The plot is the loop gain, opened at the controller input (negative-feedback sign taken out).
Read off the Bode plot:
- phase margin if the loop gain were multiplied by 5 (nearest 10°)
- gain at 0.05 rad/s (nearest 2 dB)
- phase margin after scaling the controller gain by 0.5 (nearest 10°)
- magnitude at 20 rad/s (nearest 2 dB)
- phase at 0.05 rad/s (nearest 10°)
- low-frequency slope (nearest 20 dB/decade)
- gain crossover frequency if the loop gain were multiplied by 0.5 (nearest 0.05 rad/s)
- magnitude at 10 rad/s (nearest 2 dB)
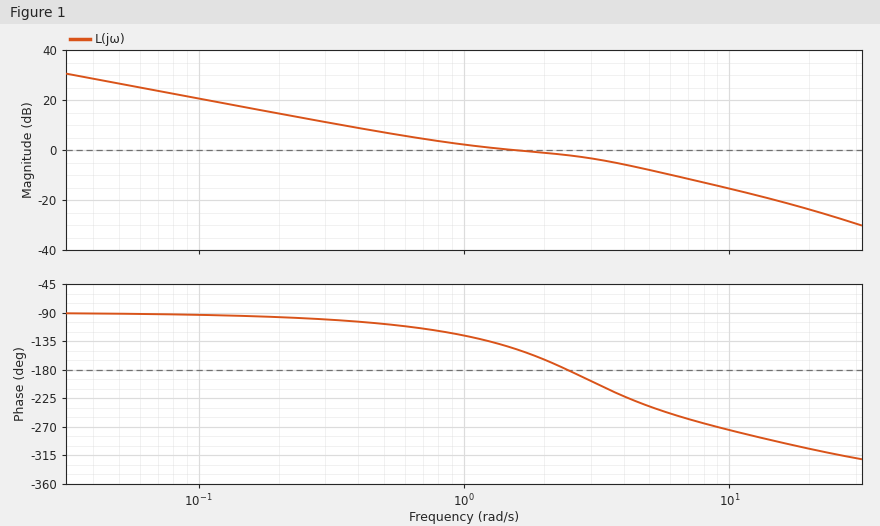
-90°
26 dB
70°
-24 dB
-90°
-20 dB/decade
0.55 rad/s
-16 dB
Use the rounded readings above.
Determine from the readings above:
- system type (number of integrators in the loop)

1
